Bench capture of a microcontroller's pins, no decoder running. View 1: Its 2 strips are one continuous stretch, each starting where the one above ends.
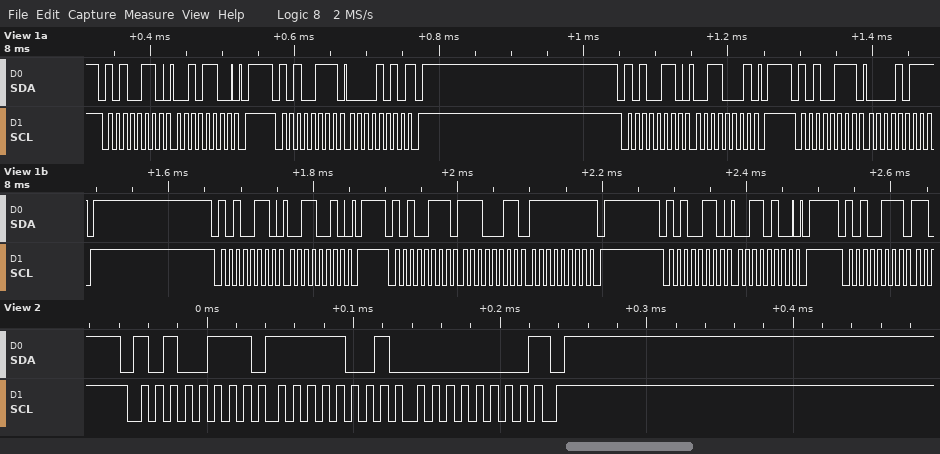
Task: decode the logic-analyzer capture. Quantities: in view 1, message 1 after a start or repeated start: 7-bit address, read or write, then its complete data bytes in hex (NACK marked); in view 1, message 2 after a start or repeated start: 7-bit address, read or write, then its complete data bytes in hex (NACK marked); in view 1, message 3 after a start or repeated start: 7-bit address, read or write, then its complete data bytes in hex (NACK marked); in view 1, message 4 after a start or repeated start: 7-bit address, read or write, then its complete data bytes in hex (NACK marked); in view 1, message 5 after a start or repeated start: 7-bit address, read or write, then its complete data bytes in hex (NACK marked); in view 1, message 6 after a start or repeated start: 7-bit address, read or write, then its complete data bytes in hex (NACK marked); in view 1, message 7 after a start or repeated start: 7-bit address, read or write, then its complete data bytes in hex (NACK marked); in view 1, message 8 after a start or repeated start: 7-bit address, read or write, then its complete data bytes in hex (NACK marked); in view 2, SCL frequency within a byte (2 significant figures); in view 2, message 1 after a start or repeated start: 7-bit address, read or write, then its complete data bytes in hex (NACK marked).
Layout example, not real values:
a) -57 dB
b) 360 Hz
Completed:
a) 0x53 write: 2C
b) 0x53 read: 0A NACK
c) 0x53 write: 31
d) 0x53 read: 0B NACK
e) 0x53 write: 32
f) 0x53 read: E3 FF NACK
g) 0x53 write: 34
h) 0x53 read
i) 100 kHz
j) 0x53 read: F9 00 NACK
